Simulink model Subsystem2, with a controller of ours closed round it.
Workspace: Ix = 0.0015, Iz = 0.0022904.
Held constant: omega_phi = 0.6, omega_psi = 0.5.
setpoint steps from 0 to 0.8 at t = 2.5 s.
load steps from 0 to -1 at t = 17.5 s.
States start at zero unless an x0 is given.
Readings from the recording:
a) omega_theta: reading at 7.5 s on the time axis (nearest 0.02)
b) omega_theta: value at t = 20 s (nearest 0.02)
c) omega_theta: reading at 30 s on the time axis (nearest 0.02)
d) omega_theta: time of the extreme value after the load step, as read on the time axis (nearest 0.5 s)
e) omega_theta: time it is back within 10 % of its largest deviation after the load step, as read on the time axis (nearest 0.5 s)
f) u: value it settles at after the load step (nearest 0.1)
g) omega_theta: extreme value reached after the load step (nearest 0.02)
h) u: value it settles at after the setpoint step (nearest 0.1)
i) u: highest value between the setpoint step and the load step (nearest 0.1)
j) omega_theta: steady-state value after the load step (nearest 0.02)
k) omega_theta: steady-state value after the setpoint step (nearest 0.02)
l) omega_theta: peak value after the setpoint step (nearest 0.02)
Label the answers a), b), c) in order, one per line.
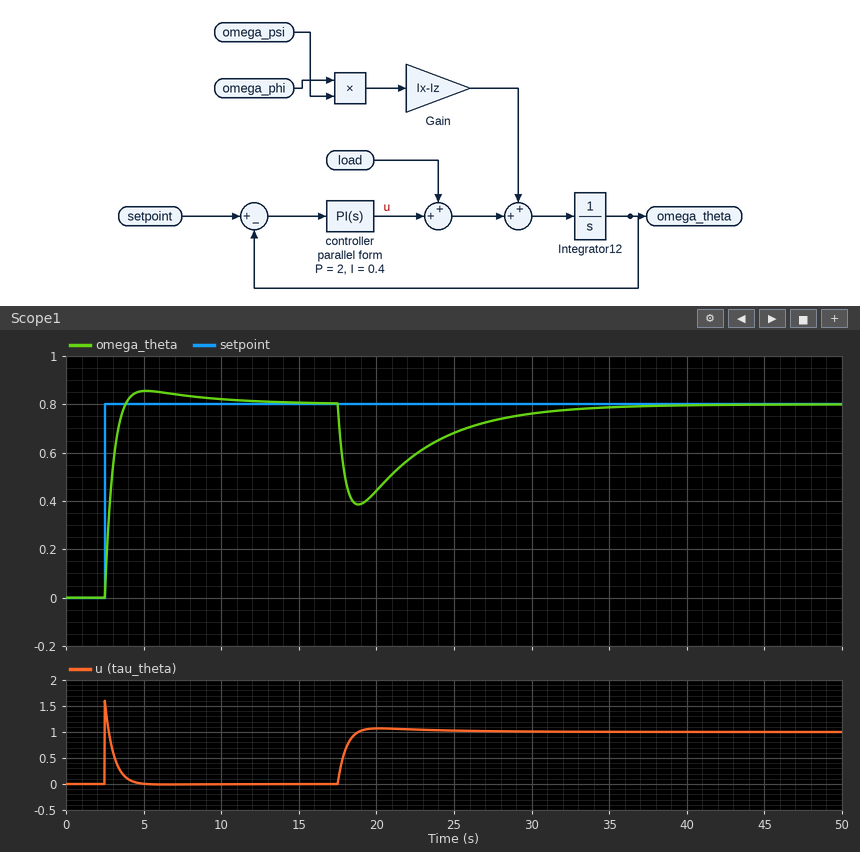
a) 0.84
b) 0.44
c) 0.76
d) 19.0 s
e) 29.5 s
f) 1.0
g) 0.38
h) 0.0
i) 1.6
j) 0.80
k) 0.80
l) 0.86
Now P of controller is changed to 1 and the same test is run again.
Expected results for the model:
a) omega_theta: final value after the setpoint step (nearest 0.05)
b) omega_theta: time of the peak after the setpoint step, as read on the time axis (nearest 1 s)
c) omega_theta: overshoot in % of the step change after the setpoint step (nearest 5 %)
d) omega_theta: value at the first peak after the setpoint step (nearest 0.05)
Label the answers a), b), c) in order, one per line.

a) 0.80
b) 6 s
c) 20 %
d) 0.95
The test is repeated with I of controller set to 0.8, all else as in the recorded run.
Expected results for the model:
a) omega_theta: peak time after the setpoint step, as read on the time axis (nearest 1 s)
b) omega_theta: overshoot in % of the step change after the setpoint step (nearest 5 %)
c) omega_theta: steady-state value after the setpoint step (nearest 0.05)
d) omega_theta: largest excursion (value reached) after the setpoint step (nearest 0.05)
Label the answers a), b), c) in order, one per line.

a) 5 s
b) 10 %
c) 0.80
d) 0.90
